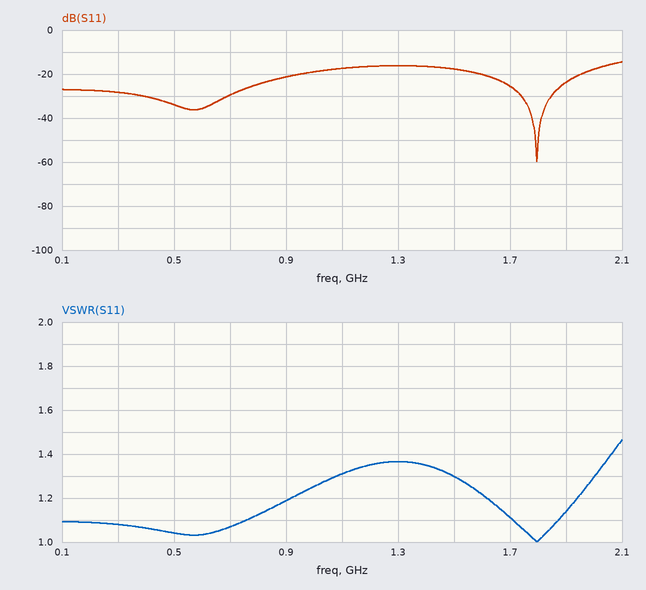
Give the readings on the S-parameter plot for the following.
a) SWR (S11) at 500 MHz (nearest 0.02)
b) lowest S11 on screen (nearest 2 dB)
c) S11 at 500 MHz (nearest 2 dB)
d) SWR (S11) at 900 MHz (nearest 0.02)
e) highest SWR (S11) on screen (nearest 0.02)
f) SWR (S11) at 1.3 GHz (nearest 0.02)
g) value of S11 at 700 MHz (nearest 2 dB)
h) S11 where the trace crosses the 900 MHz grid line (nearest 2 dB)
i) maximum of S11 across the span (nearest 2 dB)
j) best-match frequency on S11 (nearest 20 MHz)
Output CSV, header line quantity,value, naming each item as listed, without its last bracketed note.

quantity,value
SWR (S11) at 500 MHz,1.04
lowest S11 on screen,-60 dB
S11 at 500 MHz,-34 dB
SWR (S11) at 900 MHz,1.18
highest SWR (S11) on screen,1.46
SWR (S11) at 1.3 GHz,1.36
value of S11 at 700 MHz,-30 dB
S11 where the trace crosses the 900 MHz grid line,-22 dB
maximum of S11 across the span,-14 dB
best-match frequency on S11,1.80 GHz
